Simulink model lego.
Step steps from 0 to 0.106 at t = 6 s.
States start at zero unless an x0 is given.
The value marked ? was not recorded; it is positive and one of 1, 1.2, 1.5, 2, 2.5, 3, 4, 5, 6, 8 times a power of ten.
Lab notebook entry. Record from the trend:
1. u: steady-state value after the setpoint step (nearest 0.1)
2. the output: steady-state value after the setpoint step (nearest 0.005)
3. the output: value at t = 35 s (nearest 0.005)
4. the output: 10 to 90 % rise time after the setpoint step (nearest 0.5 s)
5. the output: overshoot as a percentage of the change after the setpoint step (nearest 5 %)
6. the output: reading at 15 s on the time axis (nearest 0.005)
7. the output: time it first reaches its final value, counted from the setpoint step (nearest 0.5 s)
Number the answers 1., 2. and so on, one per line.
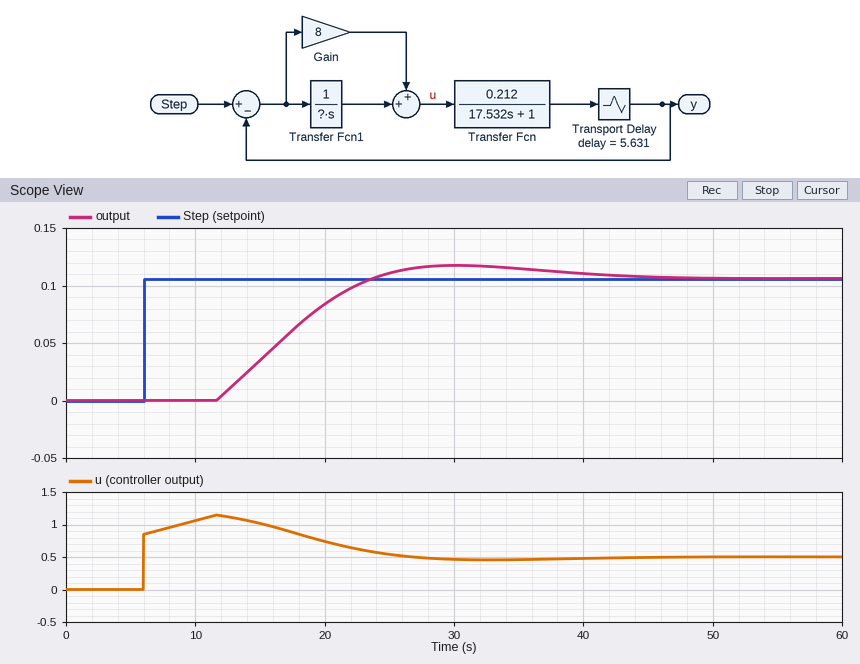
1. 0.5
2. 0.105
3. 0.115
4. 9.0 s
5. 10 %
6. 0.035
7. 17.5 s
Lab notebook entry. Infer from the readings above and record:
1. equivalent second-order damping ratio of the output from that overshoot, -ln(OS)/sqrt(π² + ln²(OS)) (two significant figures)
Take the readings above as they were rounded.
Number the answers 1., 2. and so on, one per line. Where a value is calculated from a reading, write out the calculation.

1. ln(0.1) = -2.303; 2.303 / sqrt(9.870 + 5.302) = 0.59
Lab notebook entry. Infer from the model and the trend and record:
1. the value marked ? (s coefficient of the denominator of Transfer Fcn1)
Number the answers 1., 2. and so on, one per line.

1. 2
